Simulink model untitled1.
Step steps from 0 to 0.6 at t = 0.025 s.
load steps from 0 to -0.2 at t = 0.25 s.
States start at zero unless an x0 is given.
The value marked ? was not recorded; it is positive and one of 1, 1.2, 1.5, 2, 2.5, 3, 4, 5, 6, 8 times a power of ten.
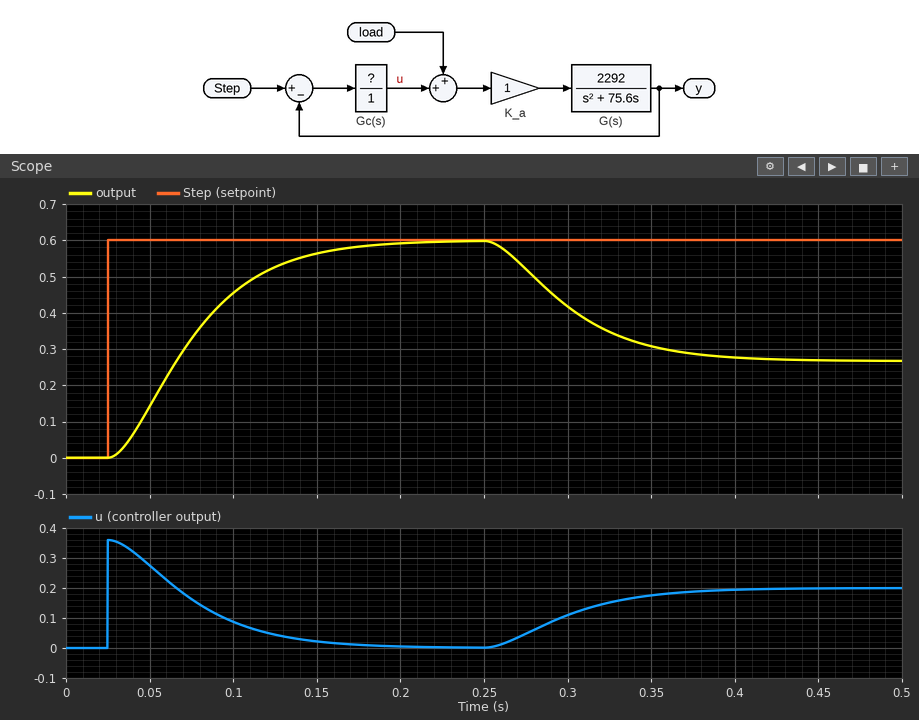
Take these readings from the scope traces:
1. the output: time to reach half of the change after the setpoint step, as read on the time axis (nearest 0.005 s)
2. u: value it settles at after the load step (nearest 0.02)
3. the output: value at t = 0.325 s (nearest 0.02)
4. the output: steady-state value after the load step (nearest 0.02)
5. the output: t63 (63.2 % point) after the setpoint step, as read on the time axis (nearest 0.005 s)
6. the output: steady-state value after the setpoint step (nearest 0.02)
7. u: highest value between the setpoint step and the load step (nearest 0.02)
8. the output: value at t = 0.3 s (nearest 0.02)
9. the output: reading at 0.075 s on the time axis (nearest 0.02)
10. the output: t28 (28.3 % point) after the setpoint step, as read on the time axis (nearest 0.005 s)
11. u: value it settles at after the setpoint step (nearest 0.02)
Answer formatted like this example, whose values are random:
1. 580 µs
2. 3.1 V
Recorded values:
1. 0.070 s
2. 0.20
3. 0.34
4. 0.26
5. 0.085 s
6. 0.60
7. 0.36
8. 0.42
9. 0.32
10. 0.055 s
11. 0.00
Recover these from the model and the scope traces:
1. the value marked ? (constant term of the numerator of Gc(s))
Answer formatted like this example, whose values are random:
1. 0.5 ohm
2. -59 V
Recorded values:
1. 0.6
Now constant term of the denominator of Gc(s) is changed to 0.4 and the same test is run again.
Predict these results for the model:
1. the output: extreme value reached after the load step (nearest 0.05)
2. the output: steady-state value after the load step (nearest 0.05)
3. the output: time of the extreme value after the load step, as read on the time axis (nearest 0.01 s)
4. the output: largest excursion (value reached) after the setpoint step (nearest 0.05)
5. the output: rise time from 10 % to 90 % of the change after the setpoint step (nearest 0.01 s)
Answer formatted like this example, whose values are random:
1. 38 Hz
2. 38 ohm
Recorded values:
1. 0.45
2. 0.45
3. 0.32 s
4. 0.65
5. 0.03 s
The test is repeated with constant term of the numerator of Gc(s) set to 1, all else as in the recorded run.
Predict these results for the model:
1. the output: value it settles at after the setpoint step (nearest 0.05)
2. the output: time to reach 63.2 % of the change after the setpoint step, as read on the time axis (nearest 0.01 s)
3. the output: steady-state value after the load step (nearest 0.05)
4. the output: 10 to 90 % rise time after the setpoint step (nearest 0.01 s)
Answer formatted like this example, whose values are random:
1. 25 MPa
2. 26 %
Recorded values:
1. 0.60
2. 0.06 s
3. 0.40
4. 0.05 s
